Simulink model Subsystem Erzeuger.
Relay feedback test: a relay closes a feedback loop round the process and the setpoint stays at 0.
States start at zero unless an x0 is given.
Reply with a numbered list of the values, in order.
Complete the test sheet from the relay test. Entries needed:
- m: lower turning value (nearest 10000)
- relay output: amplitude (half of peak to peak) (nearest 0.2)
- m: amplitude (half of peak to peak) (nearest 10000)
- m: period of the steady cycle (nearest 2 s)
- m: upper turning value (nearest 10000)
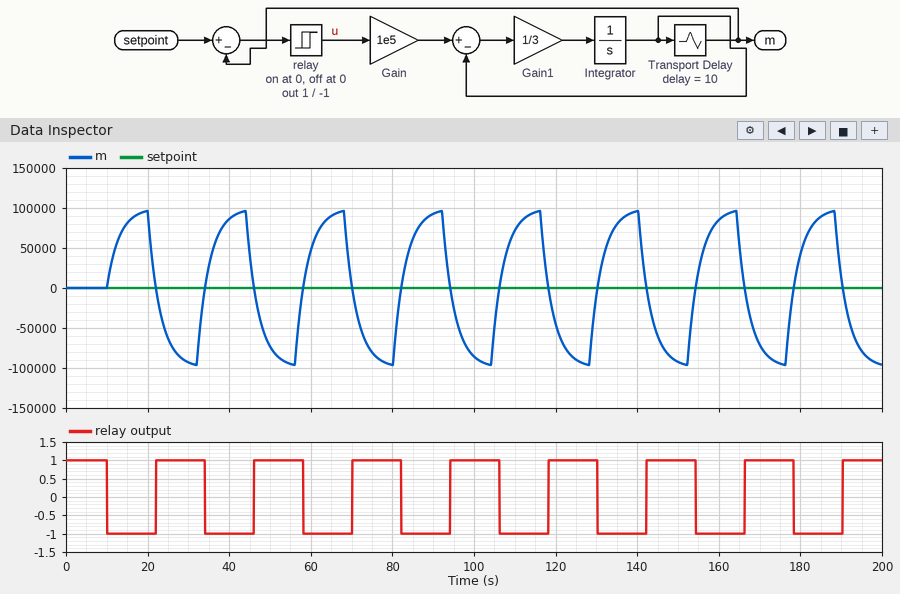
1. -100000
2. 1.0
3. 100000
4. 24 s
5. 100000
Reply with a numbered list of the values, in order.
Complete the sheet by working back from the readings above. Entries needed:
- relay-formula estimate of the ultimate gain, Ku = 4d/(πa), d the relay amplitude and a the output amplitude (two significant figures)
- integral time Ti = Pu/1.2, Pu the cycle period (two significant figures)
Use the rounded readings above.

1. 0.000013
2. 20 s
